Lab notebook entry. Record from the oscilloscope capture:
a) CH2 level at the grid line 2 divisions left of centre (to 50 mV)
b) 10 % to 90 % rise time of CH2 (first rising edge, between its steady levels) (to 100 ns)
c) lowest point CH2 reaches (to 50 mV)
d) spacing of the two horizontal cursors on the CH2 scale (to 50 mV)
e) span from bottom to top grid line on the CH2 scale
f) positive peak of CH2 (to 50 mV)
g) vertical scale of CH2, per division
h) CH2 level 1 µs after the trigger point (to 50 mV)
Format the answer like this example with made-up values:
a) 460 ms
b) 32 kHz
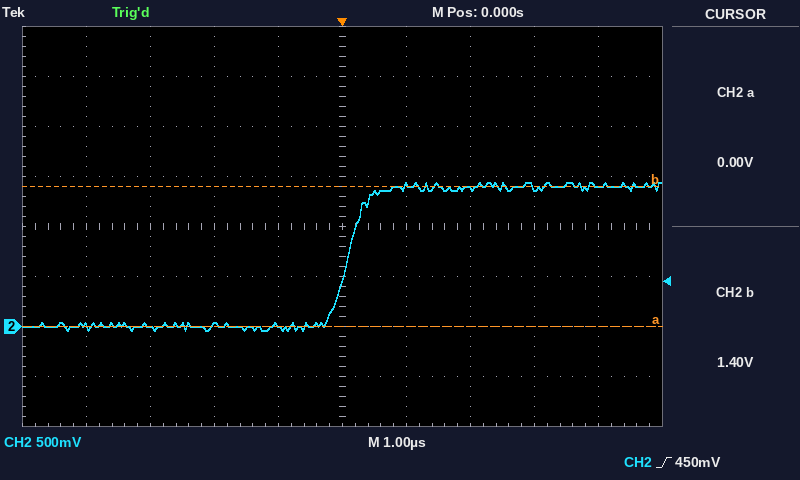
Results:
a) 0 mV
b) 600 ns
c) -50 mV
d) 1.40 V
e) 4 V
f) 1.45 V
g) 500 mV
h) 1.40 V
